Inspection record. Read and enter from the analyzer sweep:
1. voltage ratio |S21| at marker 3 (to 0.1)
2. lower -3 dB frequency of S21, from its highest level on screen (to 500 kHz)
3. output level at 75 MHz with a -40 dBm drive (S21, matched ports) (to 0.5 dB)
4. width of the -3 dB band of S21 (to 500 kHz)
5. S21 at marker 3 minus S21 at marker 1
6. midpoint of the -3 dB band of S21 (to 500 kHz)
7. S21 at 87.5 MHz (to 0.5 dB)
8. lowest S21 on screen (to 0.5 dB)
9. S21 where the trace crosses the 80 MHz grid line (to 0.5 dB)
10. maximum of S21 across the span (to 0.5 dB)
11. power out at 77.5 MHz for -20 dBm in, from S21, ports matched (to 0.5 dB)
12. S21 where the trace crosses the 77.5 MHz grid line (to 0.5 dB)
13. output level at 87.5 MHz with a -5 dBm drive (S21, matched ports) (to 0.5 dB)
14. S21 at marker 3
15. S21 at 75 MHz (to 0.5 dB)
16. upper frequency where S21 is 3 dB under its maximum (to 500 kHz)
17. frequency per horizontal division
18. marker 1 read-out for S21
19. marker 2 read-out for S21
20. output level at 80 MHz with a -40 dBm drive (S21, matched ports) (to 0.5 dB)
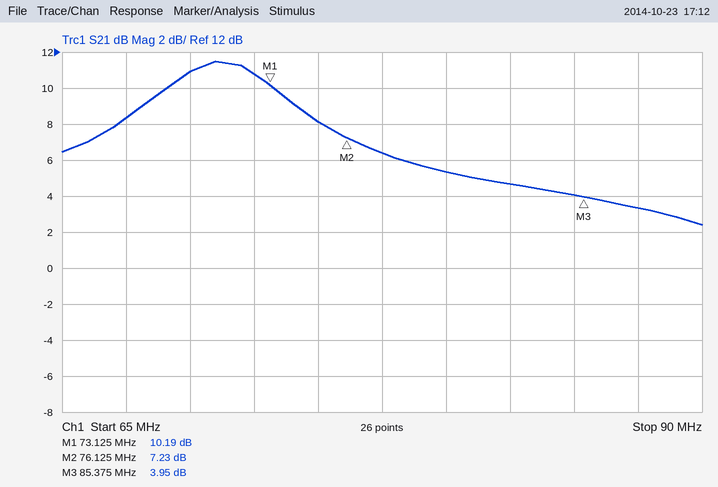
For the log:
1.6
67.5 MHz
-32.0 dBm
7.0 MHz
-6.24 dB
71.0 MHz
3.5 dB
2.5 dB
5.5 dB
11.5 dB
-13.5 dBm
6.5 dB
-1.5 dBm
3.95 dB
8.0 dB
74.5 MHz
2.5 MHz
10.19 dB
7.23 dB
-34.5 dBm
